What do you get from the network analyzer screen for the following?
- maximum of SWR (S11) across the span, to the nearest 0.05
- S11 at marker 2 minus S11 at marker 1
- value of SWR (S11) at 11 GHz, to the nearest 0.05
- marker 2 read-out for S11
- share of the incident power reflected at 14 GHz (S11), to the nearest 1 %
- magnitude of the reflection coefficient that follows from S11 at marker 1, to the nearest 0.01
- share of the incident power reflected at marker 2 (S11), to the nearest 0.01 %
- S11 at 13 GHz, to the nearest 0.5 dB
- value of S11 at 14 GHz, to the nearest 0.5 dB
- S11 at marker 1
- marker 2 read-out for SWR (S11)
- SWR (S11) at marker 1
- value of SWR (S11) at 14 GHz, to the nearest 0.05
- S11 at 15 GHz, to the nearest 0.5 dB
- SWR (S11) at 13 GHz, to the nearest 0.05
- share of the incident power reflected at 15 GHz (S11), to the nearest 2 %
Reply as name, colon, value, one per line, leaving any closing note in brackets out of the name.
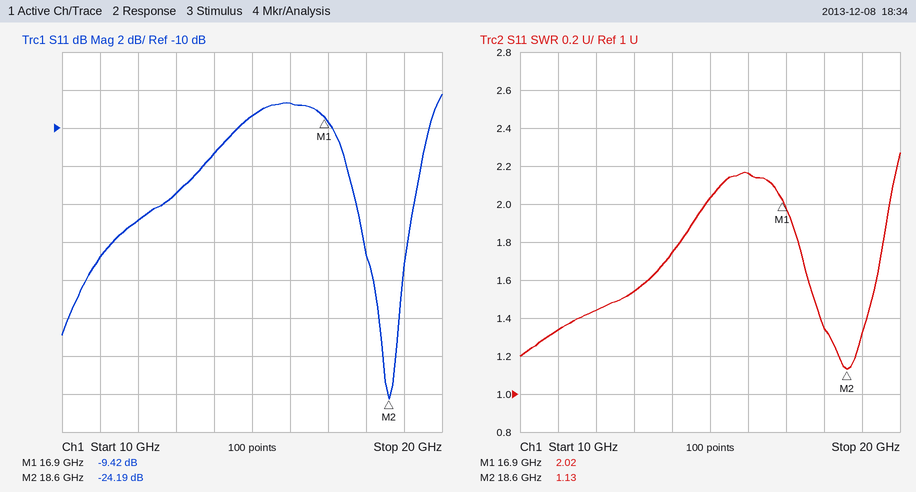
maximum of SWR (S11) across the span, to the nearest 0.05: 2.25
S11 at marker 2 minus S11 at marker 1: -14.77 dB
value of SWR (S11) at 11 GHz, to the nearest 0.05: 1.35
marker 2 read-out for S11: -24.19 dB
share of the incident power reflected at 14 GHz (S11), to the nearest 1 %: 7 %
magnitude of the reflection coefficient that follows from S11 at marker 1, to the nearest 0.01: 0.34
share of the incident power reflected at marker 2 (S11), to the nearest 0.01 %: 0.38 %
S11 at 13 GHz, to the nearest 0.5 dB: -13.5 dB
value of S11 at 14 GHz, to the nearest 0.5 dB: -11.5 dB
S11 at marker 1: -9.42 dB
marker 2 read-out for SWR: 1.13
SWR (S11) at marker 1: 2.02
value of SWR (S11) at 14 GHz, to the nearest 0.05: 1.75
S11 at 15 GHz, to the nearest 0.5 dB: -9.5 dB
SWR (S11) at 13 GHz, to the nearest 0.05: 1.55
share of the incident power reflected at 15 GHz (S11), to the nearest 2 %: 12 %
